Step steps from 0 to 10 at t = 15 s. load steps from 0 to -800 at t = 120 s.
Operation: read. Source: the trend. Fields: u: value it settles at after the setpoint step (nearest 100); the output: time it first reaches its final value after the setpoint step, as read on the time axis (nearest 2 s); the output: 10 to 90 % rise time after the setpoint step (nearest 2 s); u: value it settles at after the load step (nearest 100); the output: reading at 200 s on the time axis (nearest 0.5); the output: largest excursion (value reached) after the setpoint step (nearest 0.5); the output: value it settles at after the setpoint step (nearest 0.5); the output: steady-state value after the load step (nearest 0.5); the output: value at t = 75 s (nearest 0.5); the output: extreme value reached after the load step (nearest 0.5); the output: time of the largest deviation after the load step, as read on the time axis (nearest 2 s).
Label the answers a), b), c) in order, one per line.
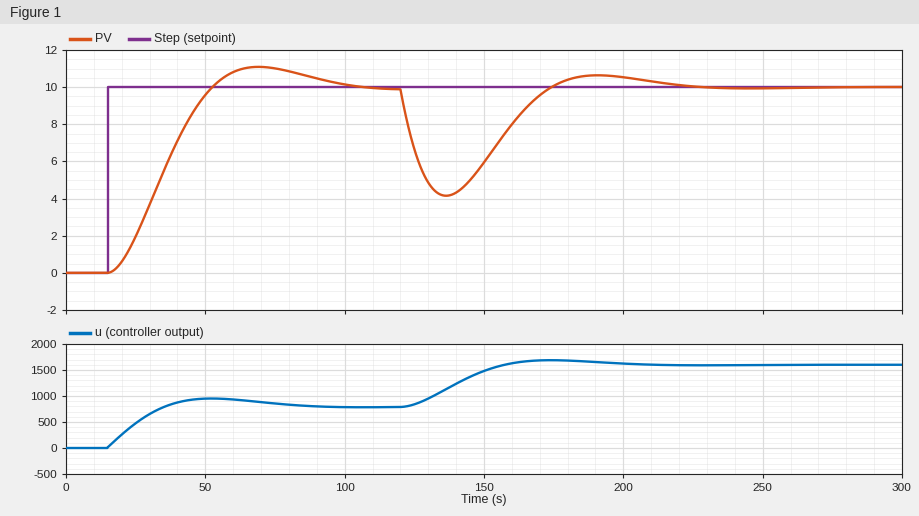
a) 800
b) 52 s
c) 26 s
d) 1600
e) 10.5
f) 11.0
g) 10.0
h) 10.0
i) 11.0
j) 4.0
k) 136 s
